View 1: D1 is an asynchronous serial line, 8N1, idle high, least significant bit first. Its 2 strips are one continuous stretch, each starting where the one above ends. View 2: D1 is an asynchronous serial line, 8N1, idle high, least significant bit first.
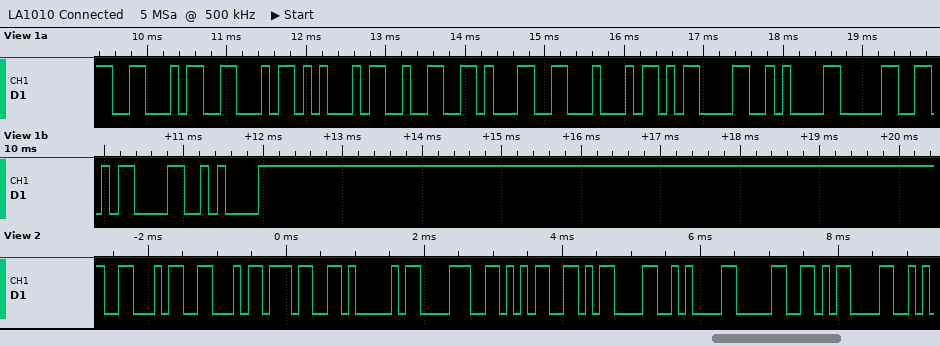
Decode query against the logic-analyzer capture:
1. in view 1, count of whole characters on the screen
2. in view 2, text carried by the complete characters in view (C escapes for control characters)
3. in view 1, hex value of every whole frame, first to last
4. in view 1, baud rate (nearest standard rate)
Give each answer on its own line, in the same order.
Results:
11
"FF7A85\r\n0\r"
0x46 0x46 0x45 0x32 0x31 0x44 0x0D 0x0A 0x30 0x0D 0x0A
9600 baud
